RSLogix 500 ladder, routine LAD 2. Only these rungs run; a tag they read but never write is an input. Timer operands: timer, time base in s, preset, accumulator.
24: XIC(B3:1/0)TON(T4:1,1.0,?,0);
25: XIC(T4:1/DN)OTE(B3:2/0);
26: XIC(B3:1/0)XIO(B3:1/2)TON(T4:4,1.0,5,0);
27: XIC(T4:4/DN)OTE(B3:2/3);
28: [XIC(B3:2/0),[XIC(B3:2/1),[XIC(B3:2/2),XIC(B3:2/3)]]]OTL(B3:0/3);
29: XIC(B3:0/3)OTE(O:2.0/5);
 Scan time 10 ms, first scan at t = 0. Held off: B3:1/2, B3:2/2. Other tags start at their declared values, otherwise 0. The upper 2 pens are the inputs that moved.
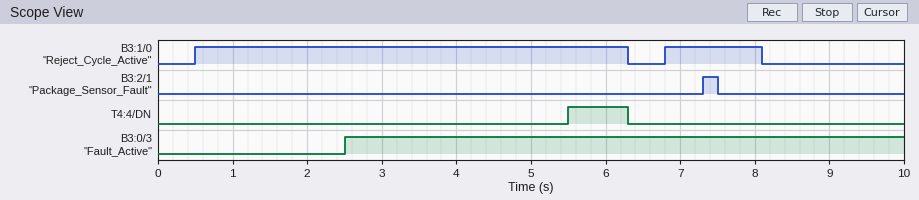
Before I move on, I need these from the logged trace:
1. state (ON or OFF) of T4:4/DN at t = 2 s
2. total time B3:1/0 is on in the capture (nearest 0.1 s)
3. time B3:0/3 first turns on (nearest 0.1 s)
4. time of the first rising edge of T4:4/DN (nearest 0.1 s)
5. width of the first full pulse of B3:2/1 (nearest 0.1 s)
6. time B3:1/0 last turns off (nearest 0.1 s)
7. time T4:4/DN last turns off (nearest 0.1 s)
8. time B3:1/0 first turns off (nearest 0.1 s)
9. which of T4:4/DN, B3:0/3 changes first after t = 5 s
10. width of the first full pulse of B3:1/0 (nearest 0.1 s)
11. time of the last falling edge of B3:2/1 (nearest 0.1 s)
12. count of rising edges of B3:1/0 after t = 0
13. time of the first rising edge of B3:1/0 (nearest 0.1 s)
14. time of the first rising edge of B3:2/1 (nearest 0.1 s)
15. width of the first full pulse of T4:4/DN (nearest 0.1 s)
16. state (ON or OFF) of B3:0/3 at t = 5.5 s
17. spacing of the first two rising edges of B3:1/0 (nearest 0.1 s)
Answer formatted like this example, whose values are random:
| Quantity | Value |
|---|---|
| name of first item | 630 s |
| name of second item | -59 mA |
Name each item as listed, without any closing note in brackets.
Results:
| Quantity | Value |
|---|---|
| state (ON or OFF) of T4:4/DN at t = 2 s | OFF |
| total time B3:1/0 is on in the capture | 7.1 s |
| time B3:0/3 first turns on | 2.5 s |
| time of the first rising edge of T4:4/DN | 5.5 s |
| width of the first full pulse of B3:2/1 | 0.2 s |
| time B3:1/0 last turns off | 8.1 s |
| time T4:4/DN last turns off | 6.3 s |
| time B3:1/0 first turns off | 6.3 s |
| which of T4:4/DN, B3:0/3 changes first after t = 5 s | T4:4/DN |
| width of the first full pulse of B3:1/0 | 5.8 s |
| time of the last falling edge of B3:2/1 | 7.5 s |
| count of rising edges of B3:1/0 after t = 0 | 2 |
| time of the first rising edge of B3:1/0 | 0.5 s |
| time of the first rising edge of B3:2/1 | 7.3 s |
| width of the first full pulse of T4:4/DN | 0.8 s |
| state (ON or OFF) of B3:0/3 at t = 5.5 s | ON |
| spacing of the first two rising edges of B3:1/0 | 6.3 s |
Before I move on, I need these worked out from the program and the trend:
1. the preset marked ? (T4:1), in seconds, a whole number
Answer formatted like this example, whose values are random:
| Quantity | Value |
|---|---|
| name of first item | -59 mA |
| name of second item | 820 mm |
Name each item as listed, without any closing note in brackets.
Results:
| Quantity | Value |
|---|---|
| the preset marked ? (T4:1), in seconds, a whole number | 2 s |
